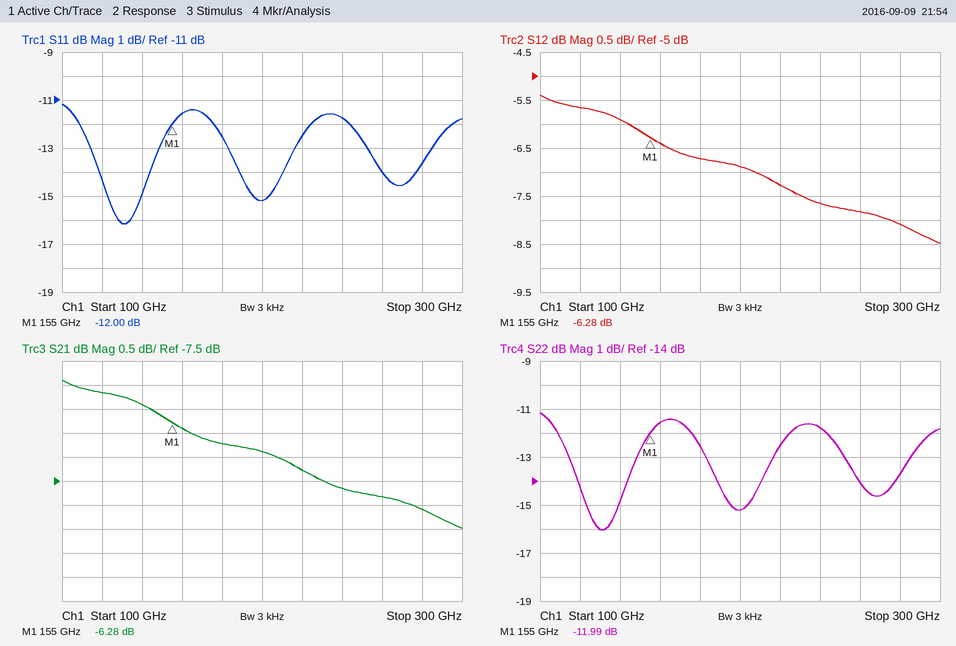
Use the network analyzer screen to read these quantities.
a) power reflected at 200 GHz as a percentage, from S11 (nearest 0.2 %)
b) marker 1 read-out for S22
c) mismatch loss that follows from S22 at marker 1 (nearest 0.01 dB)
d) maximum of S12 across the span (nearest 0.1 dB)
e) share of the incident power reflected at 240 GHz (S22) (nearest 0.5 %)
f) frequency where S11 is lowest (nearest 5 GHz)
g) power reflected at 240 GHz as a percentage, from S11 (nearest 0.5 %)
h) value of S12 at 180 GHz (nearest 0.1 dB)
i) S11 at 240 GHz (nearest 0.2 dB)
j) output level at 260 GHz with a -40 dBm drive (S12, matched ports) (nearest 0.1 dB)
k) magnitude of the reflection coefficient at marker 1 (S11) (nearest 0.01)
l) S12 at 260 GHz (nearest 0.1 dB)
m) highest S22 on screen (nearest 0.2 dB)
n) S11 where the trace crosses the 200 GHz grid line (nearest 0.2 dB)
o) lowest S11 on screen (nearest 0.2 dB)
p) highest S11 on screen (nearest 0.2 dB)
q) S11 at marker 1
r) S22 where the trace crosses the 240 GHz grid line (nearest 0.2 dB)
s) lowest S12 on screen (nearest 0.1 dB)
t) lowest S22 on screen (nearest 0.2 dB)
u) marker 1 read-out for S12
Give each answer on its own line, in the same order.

3.0 %
-11.99 dB
0.28 dB
-5.4 dB
6.5 %
130 GHz
6.5 %
-6.7 dB
-11.8 dB
-47.8 dBm
0.25
-7.8 dB
-11.2 dB
-15.2 dB
-16.2 dB
-11.2 dB
-12.00 dB
-11.8 dB
-8.5 dB
-16.0 dB
-6.28 dB
